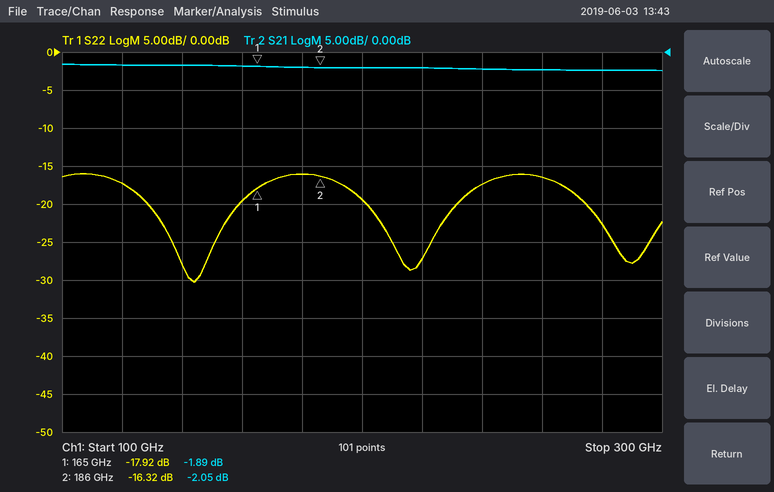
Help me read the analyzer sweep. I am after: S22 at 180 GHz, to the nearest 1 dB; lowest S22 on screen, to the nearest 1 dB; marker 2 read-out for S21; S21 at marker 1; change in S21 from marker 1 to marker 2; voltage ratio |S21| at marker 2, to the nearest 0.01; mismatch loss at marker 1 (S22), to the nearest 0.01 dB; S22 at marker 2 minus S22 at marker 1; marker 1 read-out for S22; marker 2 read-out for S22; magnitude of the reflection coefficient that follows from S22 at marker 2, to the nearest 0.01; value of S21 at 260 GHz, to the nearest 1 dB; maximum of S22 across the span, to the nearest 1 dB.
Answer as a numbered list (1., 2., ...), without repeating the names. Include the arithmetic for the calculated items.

1. -16 dB
2. -30 dB
3. -2.05 dB
4. -1.89 dB
5. -2.05 − (-1.89) = -0.16 dB
6. 10^(-2.05/20) ≈ 0.79
7. −10 log10(1 − 10^(-17.92/10)) ≈ 0.07 dB
8. -16.32 − (-17.92) = 1.60 dB
9. -17.92 dB
10. -16.32 dB
11. 10^(-16.32/20) ≈ 0.15
12. -2 dB
13. -16 dB
